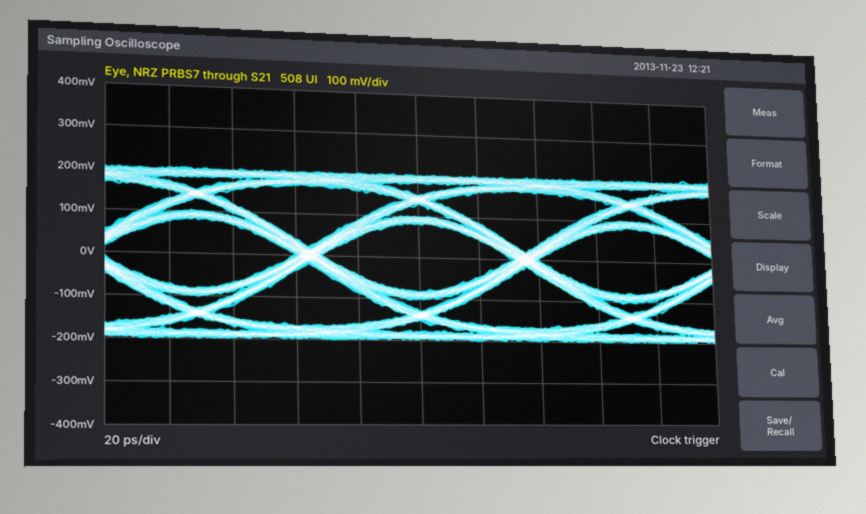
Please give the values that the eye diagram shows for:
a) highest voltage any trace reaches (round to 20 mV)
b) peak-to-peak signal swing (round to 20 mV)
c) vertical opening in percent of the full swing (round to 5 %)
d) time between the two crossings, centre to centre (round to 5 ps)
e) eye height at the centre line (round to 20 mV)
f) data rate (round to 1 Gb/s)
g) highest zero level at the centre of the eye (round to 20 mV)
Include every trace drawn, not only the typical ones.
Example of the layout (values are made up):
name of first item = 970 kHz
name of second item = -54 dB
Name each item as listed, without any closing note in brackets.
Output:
highest voltage any trace reaches = 200 mV
peak-to-peak signal swing = 400 mV
vertical opening in percent of the full swing = 40 %
time between the two crossings, centre to centre = 70 ps
eye height at the centre line = 160 mV
data rate = 14 Gb/s
highest zero level at the centre of the eye = -80 mV
